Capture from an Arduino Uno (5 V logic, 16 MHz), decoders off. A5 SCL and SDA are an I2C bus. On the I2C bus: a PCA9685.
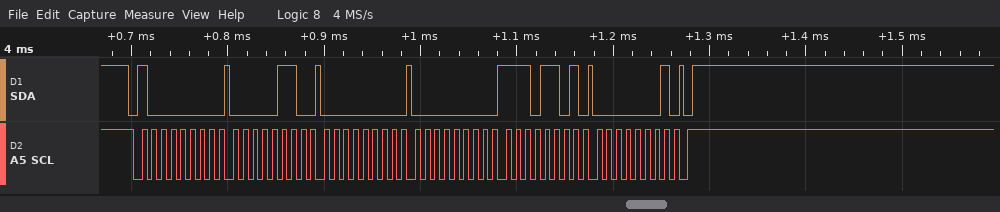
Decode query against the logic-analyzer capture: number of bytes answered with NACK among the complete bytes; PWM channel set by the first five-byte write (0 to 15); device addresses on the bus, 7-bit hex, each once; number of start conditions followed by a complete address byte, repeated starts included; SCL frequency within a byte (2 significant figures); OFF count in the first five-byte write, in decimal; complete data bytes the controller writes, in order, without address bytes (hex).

0
0
0x40
1
100 kHz
493
06 00 00 ED 01
